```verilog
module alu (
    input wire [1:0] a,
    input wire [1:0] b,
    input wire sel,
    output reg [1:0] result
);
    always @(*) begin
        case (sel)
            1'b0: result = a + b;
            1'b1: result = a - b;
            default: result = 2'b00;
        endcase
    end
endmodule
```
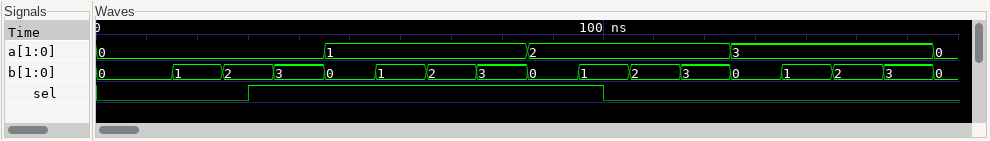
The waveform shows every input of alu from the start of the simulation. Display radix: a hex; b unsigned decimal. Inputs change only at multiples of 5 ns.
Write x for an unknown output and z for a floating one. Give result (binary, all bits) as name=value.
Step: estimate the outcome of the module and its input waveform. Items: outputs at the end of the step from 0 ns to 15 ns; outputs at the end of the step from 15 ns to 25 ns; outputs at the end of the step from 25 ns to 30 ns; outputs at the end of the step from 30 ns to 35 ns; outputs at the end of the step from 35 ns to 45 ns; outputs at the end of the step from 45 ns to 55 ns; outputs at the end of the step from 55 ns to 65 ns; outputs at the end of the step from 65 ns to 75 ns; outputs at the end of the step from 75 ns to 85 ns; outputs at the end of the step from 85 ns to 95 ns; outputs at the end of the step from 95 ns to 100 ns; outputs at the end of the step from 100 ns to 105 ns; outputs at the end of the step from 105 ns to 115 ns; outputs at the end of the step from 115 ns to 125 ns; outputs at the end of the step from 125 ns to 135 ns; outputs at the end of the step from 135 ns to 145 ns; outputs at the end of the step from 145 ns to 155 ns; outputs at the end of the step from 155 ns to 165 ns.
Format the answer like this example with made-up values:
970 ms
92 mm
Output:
result=00
result=01
result=10
result=10
result=01
result=01
result=00
result=11
result=10
result=10
result=01
result=11
result=00
result=01
result=11
result=00
result=01
result=10
